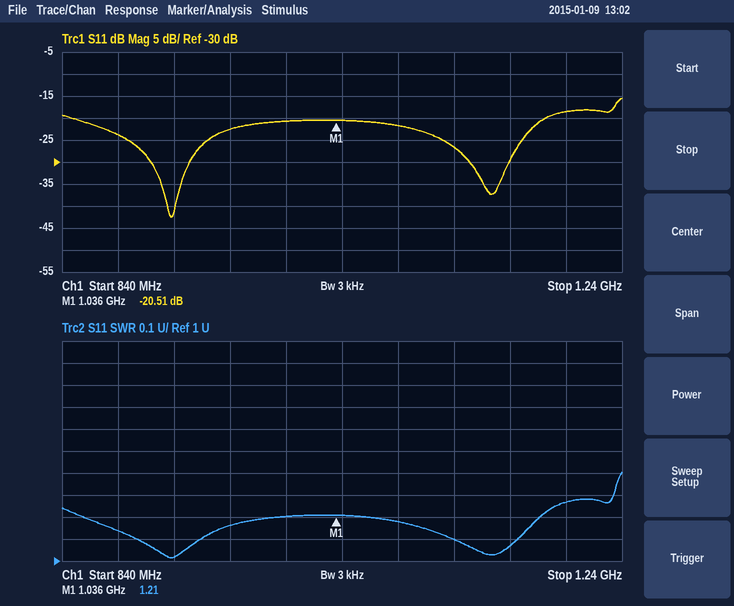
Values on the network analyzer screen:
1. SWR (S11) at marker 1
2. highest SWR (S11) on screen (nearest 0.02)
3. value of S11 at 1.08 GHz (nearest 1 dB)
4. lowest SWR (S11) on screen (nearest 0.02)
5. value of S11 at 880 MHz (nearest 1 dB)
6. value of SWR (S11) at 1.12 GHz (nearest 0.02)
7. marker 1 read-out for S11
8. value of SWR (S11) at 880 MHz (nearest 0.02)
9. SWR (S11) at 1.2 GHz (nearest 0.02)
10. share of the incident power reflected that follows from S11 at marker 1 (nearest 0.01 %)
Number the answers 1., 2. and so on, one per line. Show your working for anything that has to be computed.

1. 1.21
2. 1.40
3. -22 dB
4. 1.02
5. -24 dB
6. 1.10
7. -20.51 dB
8. 1.14
9. 1.26
10. 10^(-20.51/10) ≈ 0.89 %
